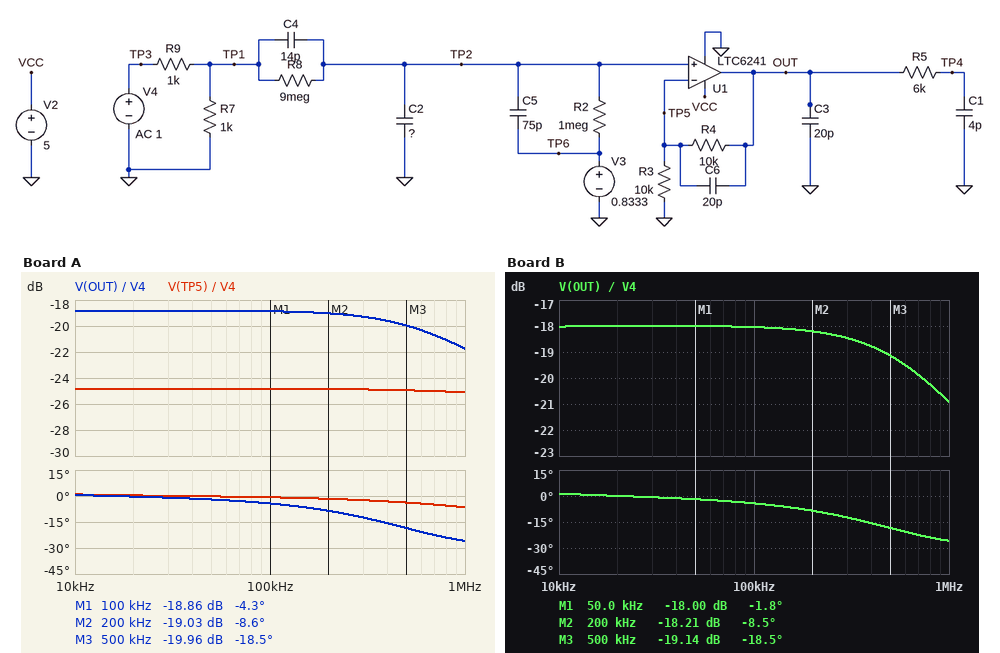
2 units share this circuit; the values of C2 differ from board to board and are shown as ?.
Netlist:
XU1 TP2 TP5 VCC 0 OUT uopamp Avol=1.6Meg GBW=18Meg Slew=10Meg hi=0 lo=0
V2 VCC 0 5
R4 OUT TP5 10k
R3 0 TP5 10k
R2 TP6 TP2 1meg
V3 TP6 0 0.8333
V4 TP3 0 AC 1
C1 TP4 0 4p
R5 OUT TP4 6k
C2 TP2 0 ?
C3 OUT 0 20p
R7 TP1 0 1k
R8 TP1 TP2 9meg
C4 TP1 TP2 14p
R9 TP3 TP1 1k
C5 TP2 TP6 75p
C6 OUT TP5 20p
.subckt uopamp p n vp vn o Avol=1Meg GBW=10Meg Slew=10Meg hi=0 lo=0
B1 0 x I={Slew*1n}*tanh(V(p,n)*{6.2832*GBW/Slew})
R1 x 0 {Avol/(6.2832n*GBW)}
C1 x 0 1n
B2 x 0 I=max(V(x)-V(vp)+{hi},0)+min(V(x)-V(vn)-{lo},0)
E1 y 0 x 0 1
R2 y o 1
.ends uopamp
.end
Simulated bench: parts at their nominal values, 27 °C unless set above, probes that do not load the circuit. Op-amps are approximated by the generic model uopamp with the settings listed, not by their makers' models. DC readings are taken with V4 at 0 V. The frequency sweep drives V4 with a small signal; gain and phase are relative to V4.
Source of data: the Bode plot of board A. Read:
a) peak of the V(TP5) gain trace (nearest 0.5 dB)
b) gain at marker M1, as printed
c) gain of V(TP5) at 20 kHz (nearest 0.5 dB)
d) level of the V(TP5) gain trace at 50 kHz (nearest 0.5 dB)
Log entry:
-25.0 dB
-18.86 dB
-25.0 dB
-25.0 dB
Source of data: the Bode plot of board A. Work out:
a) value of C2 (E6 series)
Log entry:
33 pF
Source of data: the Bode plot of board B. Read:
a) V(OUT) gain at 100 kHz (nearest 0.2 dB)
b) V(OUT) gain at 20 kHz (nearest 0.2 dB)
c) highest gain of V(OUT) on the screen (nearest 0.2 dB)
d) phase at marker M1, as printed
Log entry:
-18.0 dB
-18.0 dB
-18.0 dB
-1.8 deg
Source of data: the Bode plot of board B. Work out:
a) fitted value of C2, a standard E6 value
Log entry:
22 pF
